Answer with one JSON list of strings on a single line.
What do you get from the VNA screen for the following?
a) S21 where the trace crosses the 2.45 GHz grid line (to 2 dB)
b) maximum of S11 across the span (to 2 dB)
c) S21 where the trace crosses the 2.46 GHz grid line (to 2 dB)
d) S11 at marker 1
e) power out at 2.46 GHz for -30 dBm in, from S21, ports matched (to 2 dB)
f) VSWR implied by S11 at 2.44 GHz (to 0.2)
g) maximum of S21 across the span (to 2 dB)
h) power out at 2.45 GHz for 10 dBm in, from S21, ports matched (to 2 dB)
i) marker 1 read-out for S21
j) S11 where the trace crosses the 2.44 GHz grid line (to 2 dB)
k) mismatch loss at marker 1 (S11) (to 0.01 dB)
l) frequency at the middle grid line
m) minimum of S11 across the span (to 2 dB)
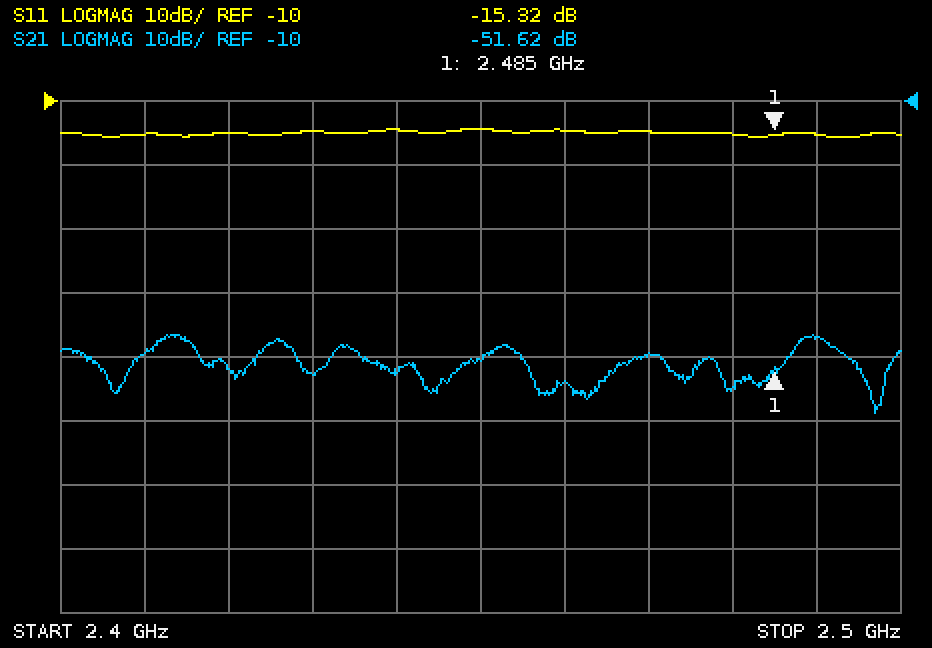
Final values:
["-50 dB", "-14 dB", "-54 dB", "-15.32 dB", "-84 dBm", "1.4", "-46 dB", "-40 dBm", "-51.62 dB", "-14 dB", "0.13 dB", "2.45 GHz", "-16 dB"]
